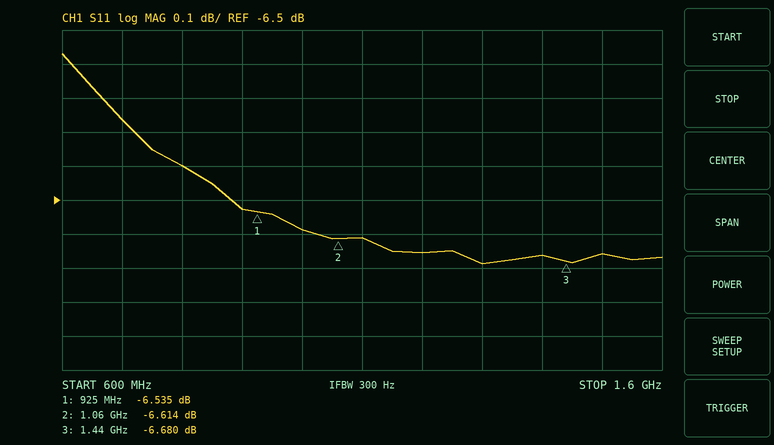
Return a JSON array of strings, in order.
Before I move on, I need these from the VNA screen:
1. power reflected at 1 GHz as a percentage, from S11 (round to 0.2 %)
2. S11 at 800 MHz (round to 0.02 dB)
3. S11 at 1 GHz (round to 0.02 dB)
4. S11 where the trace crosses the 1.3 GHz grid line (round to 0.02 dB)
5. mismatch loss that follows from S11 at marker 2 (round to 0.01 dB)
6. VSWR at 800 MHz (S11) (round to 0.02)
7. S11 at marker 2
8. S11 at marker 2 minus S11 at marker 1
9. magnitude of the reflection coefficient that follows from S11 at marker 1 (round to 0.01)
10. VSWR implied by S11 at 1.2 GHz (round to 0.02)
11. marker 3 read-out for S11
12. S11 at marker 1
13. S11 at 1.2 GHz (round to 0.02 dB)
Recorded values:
["22.0 %", "-6.40 dB", "-6.58 dB", "-6.68 dB", "1.07 dB", "2.84", "-6.614 dB", "-0.079 dB", "0.47", "2.74", "-6.680 dB", "-6.535 dB", "-6.66 dB"]
